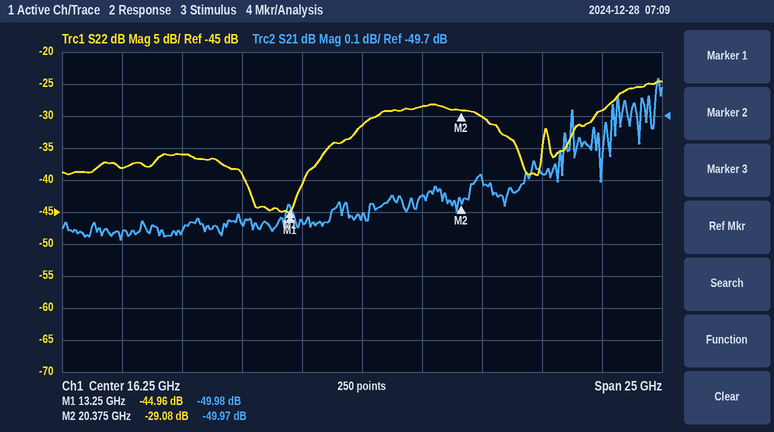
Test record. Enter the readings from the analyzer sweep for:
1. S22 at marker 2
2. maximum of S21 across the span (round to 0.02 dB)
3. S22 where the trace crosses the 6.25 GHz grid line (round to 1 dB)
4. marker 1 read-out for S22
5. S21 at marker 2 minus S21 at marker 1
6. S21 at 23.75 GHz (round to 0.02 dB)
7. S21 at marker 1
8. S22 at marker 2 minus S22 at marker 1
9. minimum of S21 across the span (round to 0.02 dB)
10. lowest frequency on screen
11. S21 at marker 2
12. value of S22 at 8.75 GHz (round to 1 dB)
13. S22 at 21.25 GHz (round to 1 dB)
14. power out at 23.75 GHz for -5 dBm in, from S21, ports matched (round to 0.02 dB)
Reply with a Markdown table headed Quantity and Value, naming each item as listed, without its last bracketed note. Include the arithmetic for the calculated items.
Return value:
| Quantity | Value |
|---|---|
| S22 at marker 2 | -29.08 dB |
| maximum of S21 across the span | -49.58 dB |
| S22 where the trace crosses the 6.25 GHz grid line | -38 dB |
| marker 1 read-out for S22 | -44.96 dB |
| S21 at marker 2 minus S21 at marker 1 | -49.97 − (-49.98) = 0.01 dB |
| S21 at 23.75 GHz | -49.88 dB |
| S21 at marker 1 | -49.98 dB |
| S22 at marker 2 minus S22 at marker 1 | -29.08 − (-44.96) = 15.88 dB |
| minimum of S21 across the span | -50.08 dB |
| lowest frequency on screen | 3.75 GHz |
| S21 at marker 2 | -49.97 dB |
| value of S22 at 8.75 GHz | -36 dB |
| S22 at 21.25 GHz | -30 dB |
| power out at 23.75 GHz for -5 dBm in, from S21, ports matched | -5 dBm + (-49.88 dB) = -54.88 dBm |
